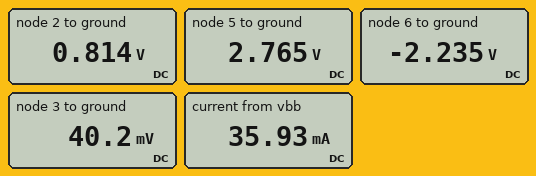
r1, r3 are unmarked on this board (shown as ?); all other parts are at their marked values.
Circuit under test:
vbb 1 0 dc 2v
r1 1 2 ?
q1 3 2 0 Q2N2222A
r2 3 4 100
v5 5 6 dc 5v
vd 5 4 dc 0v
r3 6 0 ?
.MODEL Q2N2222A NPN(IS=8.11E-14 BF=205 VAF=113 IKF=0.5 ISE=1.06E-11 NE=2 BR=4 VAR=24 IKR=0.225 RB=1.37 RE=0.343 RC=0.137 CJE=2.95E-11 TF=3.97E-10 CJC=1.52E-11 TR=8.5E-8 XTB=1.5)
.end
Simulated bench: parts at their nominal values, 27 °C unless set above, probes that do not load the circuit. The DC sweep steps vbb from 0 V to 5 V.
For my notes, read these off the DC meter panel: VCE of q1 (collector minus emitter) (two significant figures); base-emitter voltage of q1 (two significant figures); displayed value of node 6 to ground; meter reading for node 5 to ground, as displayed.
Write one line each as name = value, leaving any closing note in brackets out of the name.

VCE of q1 (collector minus emitter) = 40 mV
base-emitter voltage of q1 = 810 mV
displayed value of node 6 to ground = -2.235 V
meter reading for node 5 to ground, as displayed = 2.765 V
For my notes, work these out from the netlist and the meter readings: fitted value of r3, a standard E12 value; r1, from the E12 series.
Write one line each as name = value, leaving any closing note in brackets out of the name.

fitted value of r3, a standard E12 value = 82 Ω
r1, from the E12 series = 33 Ω
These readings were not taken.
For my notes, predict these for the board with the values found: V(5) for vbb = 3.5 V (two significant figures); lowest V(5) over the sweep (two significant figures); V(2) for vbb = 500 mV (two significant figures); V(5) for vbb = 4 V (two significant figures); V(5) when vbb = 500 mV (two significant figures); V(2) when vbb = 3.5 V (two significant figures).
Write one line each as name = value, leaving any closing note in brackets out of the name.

V(5) for vbb = 3.5 V = 2.8 V
lowest V(5) over the sweep = 2.8 V
V(2) for vbb = 500 mV = 500 mV
V(5) for vbb = 4 V = 2.8 V
V(5) when vbb = 500 mV = 5.0 V
V(2) when vbb = 3.5 V = 910 mV
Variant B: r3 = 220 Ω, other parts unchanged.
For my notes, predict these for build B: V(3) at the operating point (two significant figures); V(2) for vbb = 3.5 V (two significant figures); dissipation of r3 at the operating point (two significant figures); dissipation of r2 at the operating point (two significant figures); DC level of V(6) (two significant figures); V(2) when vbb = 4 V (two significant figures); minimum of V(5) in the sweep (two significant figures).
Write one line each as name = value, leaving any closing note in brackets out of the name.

V(3) at the operating point = 32 mV
V(2) for vbb = 3.5 V = 900 mV
dissipation of r3 at the operating point = 53 mW
dissipation of r2 at the operating point = 24 mW
DC level of V(6) = -3.4 V
V(2) when vbb = 4 V = 930 mV
minimum of V(5) in the sweep = 1.6 V
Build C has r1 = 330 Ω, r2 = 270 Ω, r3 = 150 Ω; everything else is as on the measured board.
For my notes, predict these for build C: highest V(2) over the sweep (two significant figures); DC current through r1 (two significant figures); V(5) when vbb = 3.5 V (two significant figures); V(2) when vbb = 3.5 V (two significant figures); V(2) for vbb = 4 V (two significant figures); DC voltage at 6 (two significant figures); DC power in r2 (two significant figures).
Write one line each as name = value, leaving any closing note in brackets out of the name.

highest V(2) over the sweep = 740 mV
DC current through r1 = 3.9 mA
V(5) when vbb = 3.5 V = 3.2 V
V(2) when vbb = 3.5 V = 720 mV
V(2) for vbb = 4 V = 730 mV
DC voltage at 6 = -1.8 V
DC power in r2 = 38 mW
